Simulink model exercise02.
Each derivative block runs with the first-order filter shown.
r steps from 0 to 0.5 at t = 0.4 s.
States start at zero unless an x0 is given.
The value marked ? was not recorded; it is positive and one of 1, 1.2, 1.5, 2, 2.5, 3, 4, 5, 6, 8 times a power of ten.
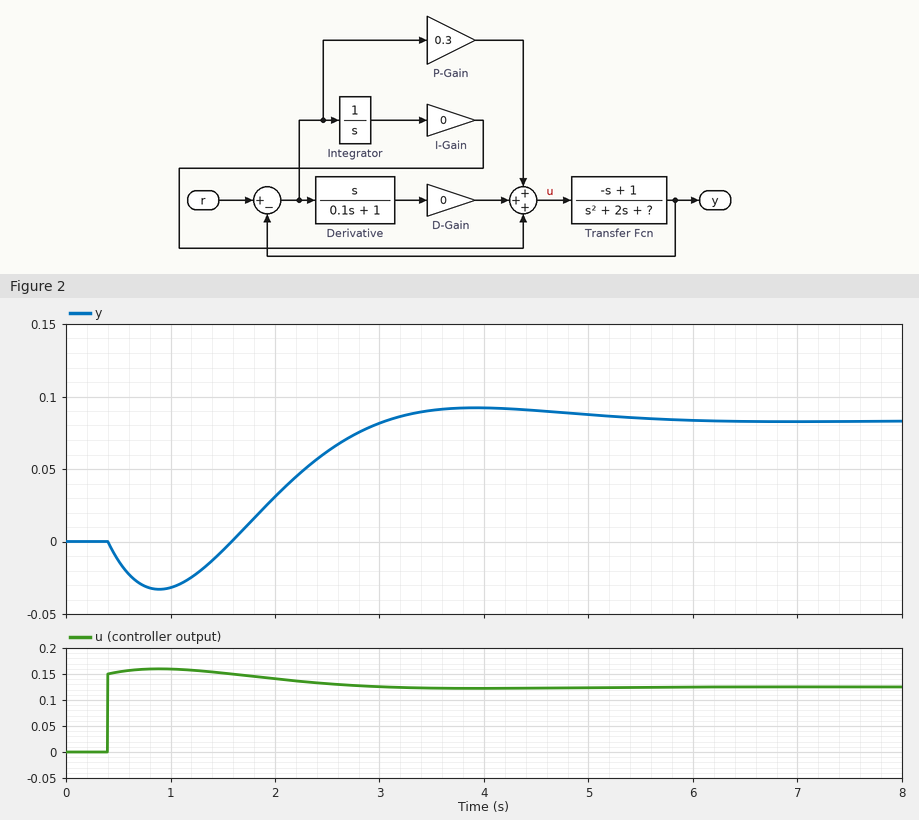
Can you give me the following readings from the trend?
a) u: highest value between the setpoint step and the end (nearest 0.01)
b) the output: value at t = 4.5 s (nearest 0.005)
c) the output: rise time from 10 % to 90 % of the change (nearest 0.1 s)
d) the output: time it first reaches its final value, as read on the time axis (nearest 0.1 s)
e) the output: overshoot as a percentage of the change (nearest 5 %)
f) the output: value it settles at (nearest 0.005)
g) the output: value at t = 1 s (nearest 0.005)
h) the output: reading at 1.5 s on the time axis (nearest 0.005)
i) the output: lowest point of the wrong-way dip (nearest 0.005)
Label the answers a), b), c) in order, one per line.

a) 0.16
b) 0.090
c) 1.1 s
d) 3.1 s
e) 10 %
f) 0.085
g) -0.030
h) -0.005
i) -0.035
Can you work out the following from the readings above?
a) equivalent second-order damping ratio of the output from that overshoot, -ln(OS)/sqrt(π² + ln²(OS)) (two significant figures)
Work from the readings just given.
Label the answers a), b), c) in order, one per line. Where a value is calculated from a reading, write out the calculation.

a) ln(0.1) = -2.303; 2.303 / sqrt(9.870 + 5.302) = 0.59
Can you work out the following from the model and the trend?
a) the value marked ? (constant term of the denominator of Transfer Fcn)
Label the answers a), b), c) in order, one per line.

a) 1.5
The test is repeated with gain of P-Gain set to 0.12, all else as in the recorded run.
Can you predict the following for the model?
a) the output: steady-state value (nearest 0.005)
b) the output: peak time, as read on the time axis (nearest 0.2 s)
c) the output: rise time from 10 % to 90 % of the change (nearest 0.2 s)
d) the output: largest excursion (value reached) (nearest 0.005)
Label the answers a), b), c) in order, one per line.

a) 0.035
b) 4.6 s
c) 1.4 s
d) 0.040
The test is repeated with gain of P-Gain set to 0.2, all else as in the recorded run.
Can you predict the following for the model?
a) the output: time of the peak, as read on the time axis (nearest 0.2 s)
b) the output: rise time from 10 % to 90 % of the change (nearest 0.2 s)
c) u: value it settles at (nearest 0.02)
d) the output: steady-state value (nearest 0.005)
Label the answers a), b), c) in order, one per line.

a) 4.2 s
b) 1.2 s
c) 0.08
d) 0.060
